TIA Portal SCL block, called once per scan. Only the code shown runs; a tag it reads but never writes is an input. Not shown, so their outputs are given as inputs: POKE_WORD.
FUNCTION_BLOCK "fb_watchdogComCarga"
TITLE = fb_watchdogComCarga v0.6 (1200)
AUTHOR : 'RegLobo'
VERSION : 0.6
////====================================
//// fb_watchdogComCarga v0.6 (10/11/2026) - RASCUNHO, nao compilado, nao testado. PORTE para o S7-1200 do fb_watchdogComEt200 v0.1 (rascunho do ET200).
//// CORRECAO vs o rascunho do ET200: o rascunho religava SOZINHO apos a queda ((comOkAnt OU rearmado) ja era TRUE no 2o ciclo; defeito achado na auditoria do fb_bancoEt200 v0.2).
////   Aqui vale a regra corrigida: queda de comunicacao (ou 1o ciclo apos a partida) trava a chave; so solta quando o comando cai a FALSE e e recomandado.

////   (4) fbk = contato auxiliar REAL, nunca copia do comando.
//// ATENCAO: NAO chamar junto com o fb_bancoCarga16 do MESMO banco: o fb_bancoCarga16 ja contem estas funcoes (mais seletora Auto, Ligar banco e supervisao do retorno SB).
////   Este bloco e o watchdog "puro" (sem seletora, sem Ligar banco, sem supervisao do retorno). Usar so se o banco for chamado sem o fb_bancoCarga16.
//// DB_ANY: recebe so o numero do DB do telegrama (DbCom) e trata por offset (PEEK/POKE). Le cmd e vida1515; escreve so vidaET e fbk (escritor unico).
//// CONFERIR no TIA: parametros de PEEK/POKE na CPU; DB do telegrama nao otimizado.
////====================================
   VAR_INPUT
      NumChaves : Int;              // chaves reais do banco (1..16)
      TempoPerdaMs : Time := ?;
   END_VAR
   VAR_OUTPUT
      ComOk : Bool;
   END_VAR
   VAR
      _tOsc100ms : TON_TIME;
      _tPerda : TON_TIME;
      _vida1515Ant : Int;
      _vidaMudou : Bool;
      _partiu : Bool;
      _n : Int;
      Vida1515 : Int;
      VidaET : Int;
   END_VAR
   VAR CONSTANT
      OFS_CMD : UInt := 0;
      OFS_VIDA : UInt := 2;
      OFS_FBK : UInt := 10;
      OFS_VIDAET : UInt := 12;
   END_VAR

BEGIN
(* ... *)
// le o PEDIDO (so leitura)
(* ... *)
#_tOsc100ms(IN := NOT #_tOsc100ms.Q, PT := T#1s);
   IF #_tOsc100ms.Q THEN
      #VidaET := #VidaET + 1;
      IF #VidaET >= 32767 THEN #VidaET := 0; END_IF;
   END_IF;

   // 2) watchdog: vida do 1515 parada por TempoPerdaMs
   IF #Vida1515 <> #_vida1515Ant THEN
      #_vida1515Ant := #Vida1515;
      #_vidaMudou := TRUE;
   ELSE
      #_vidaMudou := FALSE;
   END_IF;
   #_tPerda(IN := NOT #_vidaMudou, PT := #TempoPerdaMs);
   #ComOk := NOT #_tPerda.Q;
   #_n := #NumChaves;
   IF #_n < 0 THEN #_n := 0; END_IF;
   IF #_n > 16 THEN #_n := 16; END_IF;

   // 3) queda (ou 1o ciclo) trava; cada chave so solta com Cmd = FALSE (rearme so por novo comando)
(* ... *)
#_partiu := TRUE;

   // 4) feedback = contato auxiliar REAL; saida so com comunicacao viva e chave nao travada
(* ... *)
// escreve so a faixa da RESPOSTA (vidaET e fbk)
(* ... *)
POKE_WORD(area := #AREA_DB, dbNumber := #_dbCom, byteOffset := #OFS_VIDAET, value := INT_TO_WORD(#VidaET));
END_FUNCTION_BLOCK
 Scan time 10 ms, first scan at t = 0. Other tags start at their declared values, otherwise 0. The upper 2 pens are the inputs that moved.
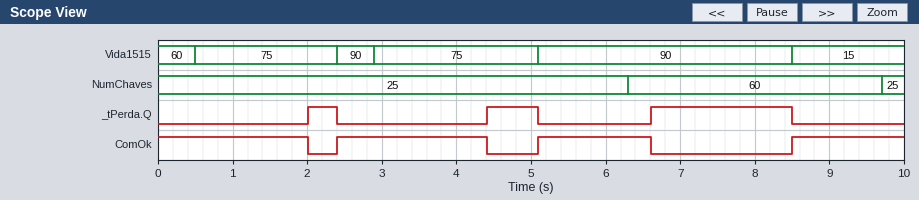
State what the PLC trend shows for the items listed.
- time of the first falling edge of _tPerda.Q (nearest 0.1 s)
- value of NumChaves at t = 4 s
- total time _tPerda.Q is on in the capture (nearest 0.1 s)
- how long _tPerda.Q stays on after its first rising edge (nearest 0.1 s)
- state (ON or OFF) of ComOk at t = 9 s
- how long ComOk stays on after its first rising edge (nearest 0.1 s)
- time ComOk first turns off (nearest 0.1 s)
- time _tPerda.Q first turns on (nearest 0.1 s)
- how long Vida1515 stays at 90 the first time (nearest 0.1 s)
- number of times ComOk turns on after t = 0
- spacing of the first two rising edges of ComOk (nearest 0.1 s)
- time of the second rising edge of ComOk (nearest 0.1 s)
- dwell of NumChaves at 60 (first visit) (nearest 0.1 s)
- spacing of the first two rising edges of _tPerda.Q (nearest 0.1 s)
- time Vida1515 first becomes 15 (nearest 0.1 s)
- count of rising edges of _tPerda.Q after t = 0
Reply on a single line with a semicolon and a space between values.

2.4 s; 25; 3.0 s; 0.4 s; ON; 2.0 s; 2.0 s; 2.0 s; 0.5 s; 3; 2.7 s; 5.1 s; 3.4 s; 2.4 s; 8.5 s; 3
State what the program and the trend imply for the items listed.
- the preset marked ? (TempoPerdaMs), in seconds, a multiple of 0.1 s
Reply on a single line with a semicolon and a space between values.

1.5 s
